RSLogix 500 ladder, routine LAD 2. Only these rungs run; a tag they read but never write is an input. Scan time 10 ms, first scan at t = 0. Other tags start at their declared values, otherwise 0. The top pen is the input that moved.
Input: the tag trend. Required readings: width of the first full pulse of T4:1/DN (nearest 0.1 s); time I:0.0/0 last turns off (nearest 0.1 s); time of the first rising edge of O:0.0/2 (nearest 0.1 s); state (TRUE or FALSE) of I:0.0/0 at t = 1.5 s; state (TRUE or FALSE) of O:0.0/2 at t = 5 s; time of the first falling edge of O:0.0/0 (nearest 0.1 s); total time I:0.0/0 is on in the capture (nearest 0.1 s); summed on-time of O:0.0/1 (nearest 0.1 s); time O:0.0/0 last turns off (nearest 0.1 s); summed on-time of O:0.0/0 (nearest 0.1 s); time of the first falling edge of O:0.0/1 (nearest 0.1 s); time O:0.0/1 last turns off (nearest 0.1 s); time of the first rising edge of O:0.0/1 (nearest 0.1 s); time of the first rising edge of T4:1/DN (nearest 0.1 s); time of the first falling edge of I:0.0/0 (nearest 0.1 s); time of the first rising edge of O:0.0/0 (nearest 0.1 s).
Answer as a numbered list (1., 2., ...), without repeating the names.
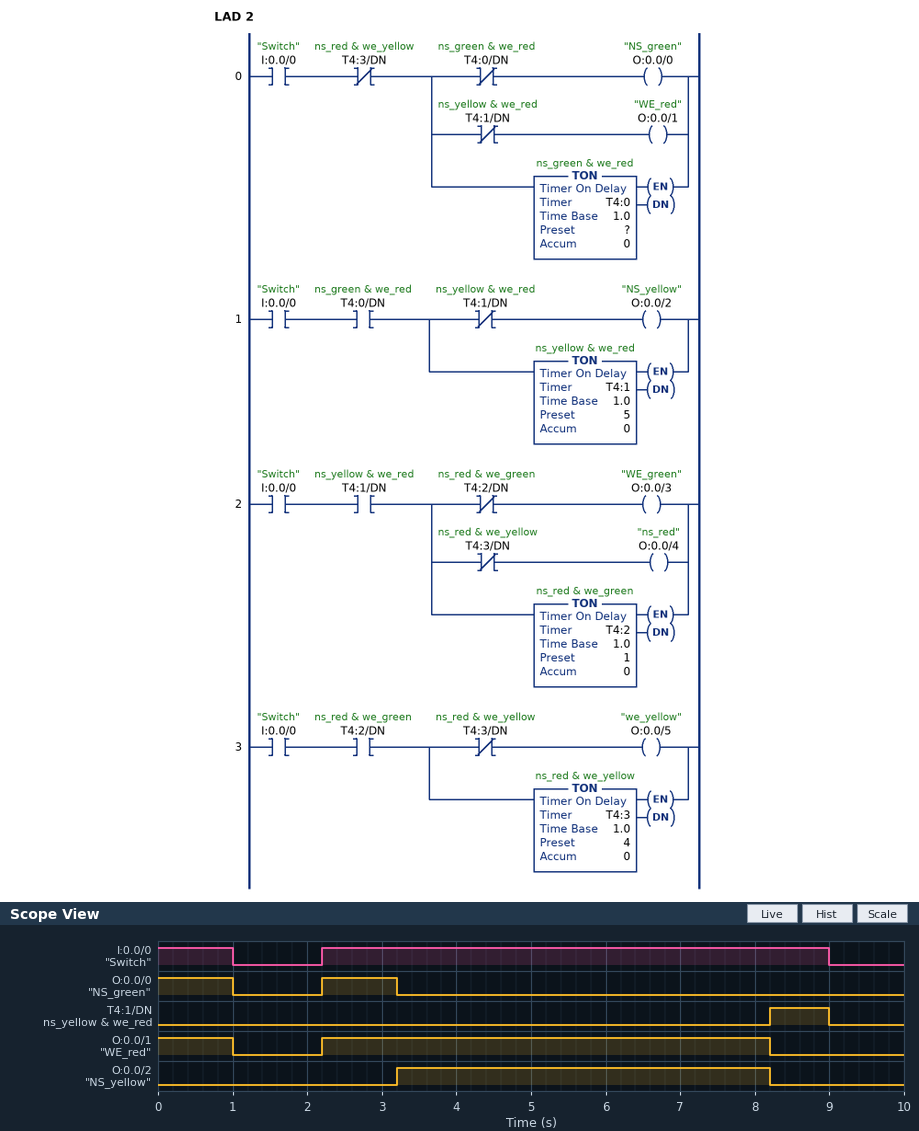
1. 0.8 s
2. 9.0 s
3. 3.2 s
4. FALSE
5. TRUE
6. 1.0 s
7. 7.8 s
8. 7.0 s
9. 3.2 s
10. 2.0 s
11. 1.0 s
12. 8.2 s
13. 2.2 s
14. 8.2 s
15. 1.0 s
16. 2.2 s
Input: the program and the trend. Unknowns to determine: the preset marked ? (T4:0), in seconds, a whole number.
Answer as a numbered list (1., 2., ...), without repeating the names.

1. 1 s
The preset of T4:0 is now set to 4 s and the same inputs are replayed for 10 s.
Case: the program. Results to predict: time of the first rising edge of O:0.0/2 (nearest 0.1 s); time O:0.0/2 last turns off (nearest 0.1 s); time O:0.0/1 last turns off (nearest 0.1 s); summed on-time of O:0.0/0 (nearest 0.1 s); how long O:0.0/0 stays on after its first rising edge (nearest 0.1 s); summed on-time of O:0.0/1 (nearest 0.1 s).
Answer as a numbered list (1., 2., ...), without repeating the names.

1. 6.2 s
2. 9.0 s
3. 9.0 s
4. 5.0 s
5. 4.0 s
6. 7.8 s
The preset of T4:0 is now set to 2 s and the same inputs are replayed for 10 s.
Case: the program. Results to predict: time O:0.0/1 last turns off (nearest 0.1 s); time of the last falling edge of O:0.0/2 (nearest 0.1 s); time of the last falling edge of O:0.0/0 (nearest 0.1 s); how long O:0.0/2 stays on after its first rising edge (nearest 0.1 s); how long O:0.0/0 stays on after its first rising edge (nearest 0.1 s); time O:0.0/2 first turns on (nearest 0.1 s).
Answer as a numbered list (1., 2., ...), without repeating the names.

1. 9.0 s
2. 9.0 s
3. 4.2 s
4. 4.8 s
5. 2.0 s
6. 4.2 s
